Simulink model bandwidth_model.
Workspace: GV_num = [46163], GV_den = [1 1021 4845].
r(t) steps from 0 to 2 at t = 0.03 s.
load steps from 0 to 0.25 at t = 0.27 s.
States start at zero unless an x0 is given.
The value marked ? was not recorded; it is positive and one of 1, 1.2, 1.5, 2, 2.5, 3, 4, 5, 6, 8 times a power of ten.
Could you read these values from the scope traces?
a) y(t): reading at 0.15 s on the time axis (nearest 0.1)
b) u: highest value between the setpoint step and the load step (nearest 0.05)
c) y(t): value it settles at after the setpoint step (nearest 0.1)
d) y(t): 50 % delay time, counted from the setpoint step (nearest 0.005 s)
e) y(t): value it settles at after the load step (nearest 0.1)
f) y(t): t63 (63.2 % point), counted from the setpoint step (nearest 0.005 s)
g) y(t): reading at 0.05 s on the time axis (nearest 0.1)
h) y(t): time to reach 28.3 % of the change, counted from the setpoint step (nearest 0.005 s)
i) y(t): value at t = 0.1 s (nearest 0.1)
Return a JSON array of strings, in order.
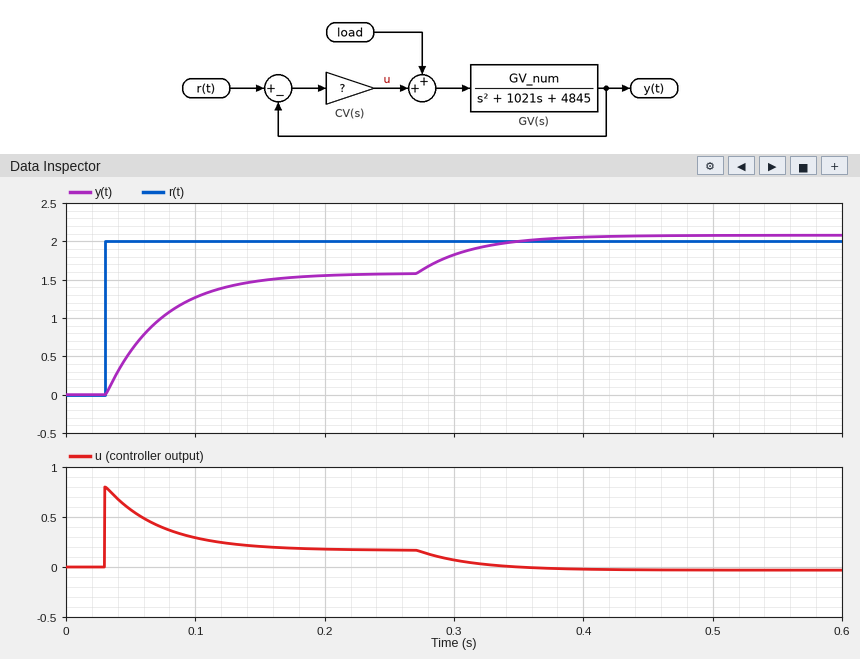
["1.5", "0.80", "1.6", "0.030 s", "2.1", "0.045 s", "0.6", "0.015 s", "1.3"]
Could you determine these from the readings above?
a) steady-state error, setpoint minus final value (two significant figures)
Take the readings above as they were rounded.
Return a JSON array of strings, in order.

["0.40"]
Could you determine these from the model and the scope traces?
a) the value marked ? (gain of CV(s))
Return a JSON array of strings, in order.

["0.4"]
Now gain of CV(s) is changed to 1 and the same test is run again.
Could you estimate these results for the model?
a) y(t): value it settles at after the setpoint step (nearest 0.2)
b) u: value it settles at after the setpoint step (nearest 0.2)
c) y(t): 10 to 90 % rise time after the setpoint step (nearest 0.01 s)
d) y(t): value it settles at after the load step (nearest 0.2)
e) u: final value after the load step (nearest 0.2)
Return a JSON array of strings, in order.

["1.8", "0.2", "0.04 s", "2.0", "0.0"]
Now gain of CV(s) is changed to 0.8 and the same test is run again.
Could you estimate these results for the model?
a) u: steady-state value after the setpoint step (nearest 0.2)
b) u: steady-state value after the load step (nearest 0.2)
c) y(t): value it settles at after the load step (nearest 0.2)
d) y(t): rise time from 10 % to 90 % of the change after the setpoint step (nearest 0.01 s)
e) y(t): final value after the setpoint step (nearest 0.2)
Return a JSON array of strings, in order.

["0.2", "0.0", "2.0", "0.05 s", "1.8"]
